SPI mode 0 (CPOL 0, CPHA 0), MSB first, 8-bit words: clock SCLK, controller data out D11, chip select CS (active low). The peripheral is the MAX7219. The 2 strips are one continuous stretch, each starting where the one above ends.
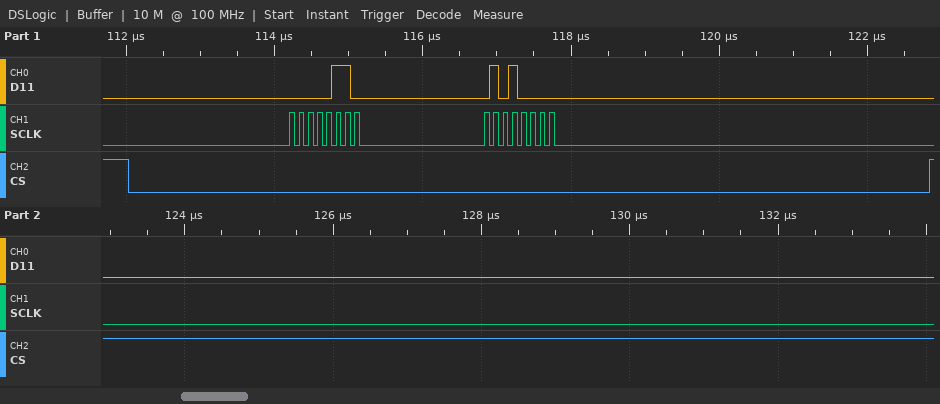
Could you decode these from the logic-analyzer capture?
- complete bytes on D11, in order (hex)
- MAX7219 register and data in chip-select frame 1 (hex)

06 50
register 0x6, data 0x50
